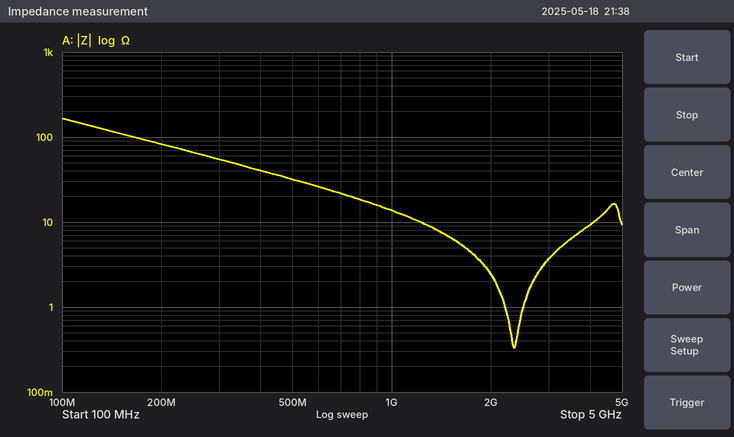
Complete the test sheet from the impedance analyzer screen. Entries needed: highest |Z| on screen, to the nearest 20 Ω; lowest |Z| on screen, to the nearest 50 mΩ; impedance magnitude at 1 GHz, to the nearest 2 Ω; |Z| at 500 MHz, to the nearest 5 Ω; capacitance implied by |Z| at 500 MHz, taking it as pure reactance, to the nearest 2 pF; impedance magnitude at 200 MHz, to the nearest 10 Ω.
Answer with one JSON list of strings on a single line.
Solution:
["160 Ω", "350 mΩ", "14 Ω", "30 Ω", "10 pF", "80 Ω"]
